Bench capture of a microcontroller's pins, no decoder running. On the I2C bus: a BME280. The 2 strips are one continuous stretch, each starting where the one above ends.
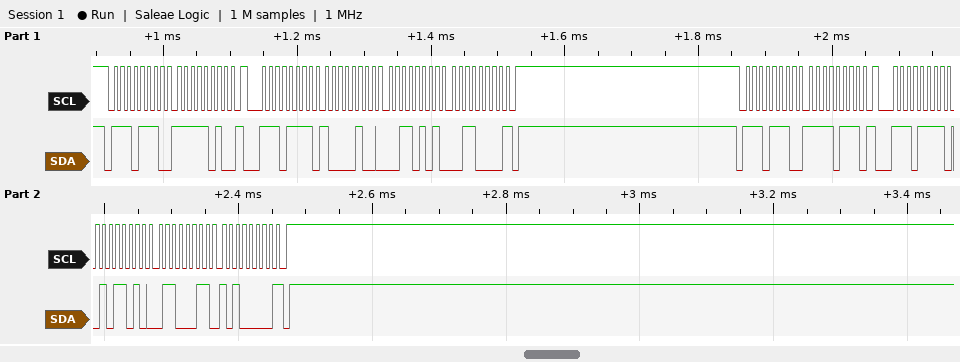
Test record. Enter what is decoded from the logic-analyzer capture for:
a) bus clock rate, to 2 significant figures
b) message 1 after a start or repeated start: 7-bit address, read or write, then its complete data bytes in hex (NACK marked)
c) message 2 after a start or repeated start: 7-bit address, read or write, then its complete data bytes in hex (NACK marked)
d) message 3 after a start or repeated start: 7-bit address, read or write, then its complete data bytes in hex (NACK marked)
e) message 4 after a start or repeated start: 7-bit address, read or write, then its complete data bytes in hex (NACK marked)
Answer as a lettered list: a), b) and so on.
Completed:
a) 100 kHz
b) 0x77 write: FA
c) 0x77 read: 84 35 30 NACK
d) 0x77 write: F7
e) 0x77 read: 5A 63 A0 NACK
